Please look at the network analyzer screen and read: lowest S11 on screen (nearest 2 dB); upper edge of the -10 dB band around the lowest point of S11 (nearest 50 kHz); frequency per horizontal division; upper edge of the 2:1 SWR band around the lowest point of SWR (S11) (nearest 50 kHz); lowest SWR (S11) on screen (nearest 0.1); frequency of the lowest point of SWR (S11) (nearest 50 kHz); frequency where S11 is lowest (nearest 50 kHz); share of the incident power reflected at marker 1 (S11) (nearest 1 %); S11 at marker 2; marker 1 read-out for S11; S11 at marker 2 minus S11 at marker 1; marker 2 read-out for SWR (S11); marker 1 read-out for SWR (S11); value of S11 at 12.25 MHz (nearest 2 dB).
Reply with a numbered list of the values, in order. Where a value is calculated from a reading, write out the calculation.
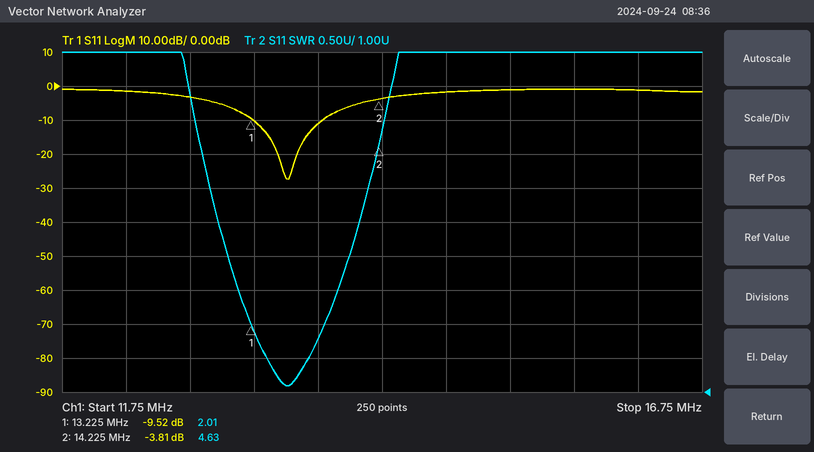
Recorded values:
1. -28 dB
2. 13.80 MHz
3. 500 kHz
4. 13.80 MHz
5. 1.1
6. 13.50 MHz
7. 13.50 MHz
8. 10^(-9.52/10) ≈ 11 %
9. -3.81 dB
10. -9.52 dB
11. -3.81 − (-9.52) = 5.71 dB
12. 4.63
13. 2.01
14. -2 dB
